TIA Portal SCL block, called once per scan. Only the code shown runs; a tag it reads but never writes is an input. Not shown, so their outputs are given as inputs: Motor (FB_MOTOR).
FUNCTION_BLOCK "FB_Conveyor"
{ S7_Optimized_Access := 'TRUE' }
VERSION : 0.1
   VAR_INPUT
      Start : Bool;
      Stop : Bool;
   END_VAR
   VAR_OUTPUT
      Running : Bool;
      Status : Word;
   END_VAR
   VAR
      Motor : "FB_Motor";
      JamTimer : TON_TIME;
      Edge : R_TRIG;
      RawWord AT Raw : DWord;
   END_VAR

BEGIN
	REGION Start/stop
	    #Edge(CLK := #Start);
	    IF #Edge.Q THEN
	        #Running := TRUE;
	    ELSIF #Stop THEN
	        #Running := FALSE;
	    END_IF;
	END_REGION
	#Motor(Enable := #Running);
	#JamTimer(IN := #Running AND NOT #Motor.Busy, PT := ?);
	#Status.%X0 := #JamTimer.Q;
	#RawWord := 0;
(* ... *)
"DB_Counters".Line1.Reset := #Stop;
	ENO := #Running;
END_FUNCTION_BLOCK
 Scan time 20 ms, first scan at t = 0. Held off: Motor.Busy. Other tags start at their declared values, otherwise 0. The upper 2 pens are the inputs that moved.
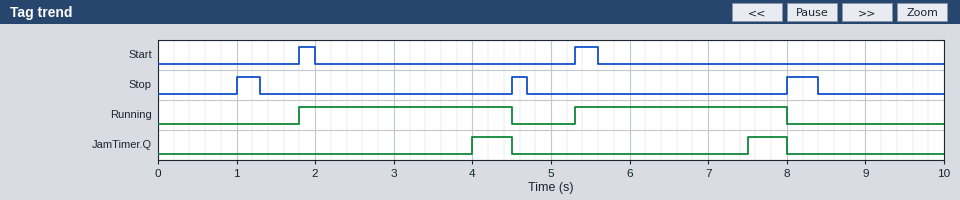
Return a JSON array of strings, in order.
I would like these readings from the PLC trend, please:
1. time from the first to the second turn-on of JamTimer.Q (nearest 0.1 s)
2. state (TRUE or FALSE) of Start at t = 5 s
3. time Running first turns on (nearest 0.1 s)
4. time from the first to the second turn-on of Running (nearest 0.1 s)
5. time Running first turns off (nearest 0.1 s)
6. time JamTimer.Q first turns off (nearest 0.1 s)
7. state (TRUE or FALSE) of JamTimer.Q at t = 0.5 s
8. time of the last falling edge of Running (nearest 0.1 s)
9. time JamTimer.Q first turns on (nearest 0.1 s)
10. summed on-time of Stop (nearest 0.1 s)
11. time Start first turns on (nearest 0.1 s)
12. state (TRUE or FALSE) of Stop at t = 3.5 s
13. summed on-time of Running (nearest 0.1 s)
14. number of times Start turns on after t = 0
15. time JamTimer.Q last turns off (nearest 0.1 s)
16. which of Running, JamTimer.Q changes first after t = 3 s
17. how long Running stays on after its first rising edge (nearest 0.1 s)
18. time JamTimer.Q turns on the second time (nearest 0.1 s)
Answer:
["3.5 s", "FALSE", "1.8 s", "3.5 s", "4.5 s", "4.5 s", "FALSE", "8.0 s", "4.0 s", "0.9 s", "1.8 s", "FALSE", "5.4 s", "2", "8.0 s", "JamTimer.Q", "2.7 s", "7.5 s"]
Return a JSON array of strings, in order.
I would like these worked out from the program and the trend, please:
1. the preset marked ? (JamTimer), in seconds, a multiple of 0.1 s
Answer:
["2.2 s"]
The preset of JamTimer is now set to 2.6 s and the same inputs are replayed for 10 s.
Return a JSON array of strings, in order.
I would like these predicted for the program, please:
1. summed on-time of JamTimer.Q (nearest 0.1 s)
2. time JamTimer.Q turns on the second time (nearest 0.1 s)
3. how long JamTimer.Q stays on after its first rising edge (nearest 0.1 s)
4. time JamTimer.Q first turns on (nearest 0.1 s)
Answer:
["0.2 s", "7.9 s", "0.1 s", "4.4 s"]
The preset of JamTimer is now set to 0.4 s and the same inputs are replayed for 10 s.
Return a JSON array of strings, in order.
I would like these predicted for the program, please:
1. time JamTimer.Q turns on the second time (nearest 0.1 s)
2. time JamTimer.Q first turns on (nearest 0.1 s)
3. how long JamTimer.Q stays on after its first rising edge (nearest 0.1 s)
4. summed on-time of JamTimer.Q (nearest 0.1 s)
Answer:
["5.7 s", "2.2 s", "2.3 s", "4.6 s"]
